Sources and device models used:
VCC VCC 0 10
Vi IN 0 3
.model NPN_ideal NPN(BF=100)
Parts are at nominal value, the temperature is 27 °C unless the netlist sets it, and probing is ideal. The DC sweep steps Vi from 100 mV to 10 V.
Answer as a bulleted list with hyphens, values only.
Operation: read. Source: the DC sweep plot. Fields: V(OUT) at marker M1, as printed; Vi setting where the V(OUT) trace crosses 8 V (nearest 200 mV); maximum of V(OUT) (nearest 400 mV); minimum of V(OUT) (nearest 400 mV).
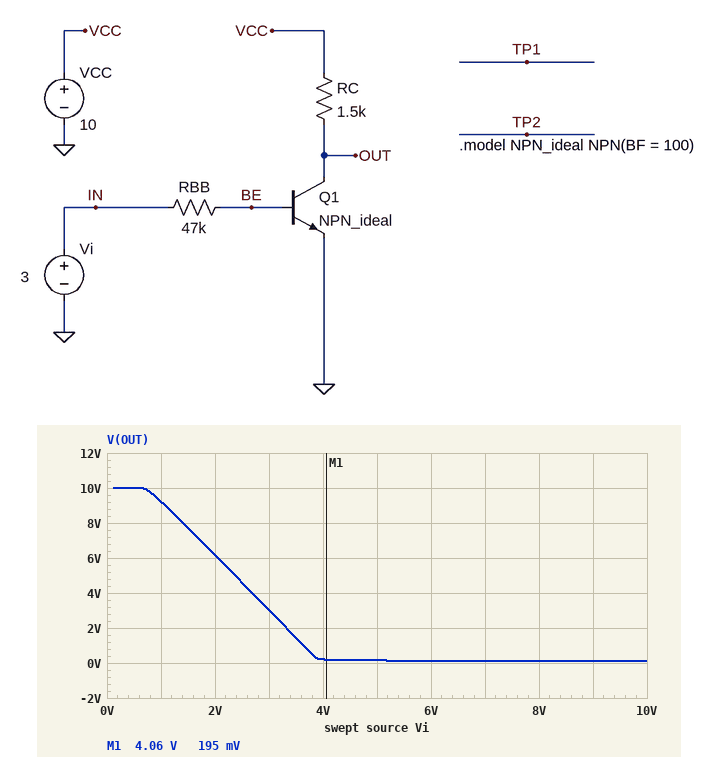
- 195 mV
- 1.4 V
- 10.0 V
- 0 V
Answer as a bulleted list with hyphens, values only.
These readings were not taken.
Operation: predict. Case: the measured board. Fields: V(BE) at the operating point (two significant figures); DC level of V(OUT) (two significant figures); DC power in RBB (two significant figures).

- 810 mV
- 3.0 V
- 100 µW
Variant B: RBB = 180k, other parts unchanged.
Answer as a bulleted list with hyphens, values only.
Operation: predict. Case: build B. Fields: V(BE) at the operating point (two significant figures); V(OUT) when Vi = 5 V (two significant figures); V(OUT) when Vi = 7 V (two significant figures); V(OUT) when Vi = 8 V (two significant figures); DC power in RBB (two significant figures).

- 780 mV
- 6.5 V
- 4.8 V
- 4.0 V
- 27 µW
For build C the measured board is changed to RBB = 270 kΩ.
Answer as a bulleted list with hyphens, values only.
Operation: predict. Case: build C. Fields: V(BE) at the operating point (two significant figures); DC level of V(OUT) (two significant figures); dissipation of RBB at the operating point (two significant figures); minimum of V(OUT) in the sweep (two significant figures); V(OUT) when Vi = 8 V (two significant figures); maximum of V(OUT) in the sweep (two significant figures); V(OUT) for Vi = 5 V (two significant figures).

- 770 mV
- 8.8 V
- 18 µW
- 4.9 V
- 6.0 V
- 10 V
- 7.7 V
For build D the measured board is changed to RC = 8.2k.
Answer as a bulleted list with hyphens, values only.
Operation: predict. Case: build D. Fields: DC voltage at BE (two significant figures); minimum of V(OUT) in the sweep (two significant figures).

- 780 mV
- 56 mV
